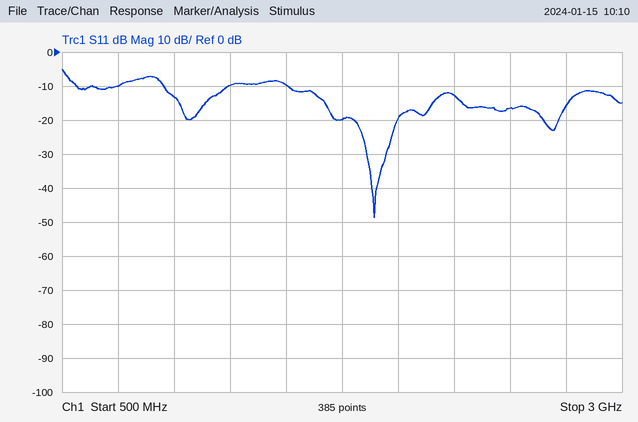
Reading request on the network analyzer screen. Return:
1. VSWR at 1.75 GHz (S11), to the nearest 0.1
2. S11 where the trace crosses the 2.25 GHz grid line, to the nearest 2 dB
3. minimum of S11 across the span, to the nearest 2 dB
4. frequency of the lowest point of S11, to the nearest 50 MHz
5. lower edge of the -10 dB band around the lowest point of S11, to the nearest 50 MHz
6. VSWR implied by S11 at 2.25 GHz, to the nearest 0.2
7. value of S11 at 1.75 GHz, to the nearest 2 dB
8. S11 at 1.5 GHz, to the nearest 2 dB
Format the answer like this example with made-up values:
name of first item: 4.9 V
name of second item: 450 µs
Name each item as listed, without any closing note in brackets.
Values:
VSWR at 1.75 GHz (S11), to the nearest 0.1: 1.2
S11 where the trace crosses the 2.25 GHz grid line, to the nearest 2 dB: -12 dB
minimum of S11 across the span, to the nearest 2 dB: -48 dB
frequency of the lowest point of S11, to the nearest 50 MHz: 1.90 GHz
lower edge of the -10 dB band around the lowest point of S11, to the nearest 50 MHz: 1.50 GHz
VSWR implied by S11 at 2.25 GHz, to the nearest 0.2: 1.6
value of S11 at 1.75 GHz, to the nearest 2 dB: -20 dB
S11 at 1.5 GHz, to the nearest 2 dB: -10 dB
